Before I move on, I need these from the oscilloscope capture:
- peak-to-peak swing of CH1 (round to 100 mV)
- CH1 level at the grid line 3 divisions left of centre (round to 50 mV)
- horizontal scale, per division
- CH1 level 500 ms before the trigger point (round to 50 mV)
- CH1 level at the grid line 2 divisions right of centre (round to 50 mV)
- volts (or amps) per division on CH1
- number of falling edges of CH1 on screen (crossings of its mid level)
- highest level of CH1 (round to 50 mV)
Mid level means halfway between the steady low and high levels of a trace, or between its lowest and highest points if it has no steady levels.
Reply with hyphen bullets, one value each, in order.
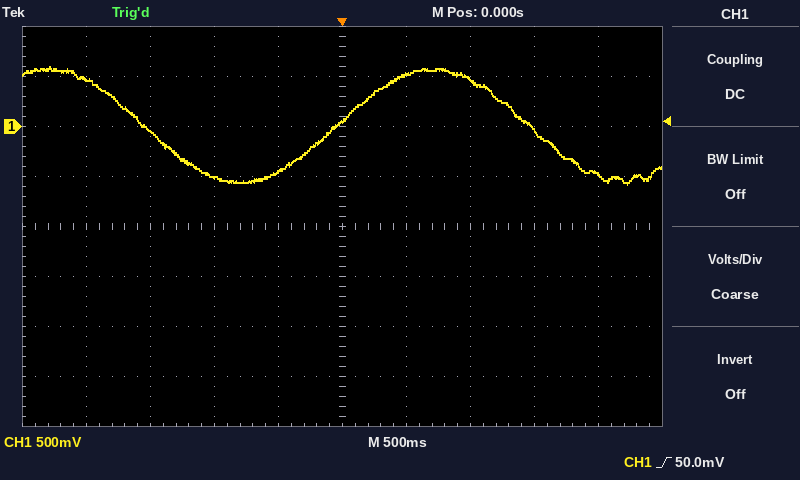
- 1.20 V
- -50 mV
- 500 ms
- -450 mV
- 450 mV
- 500 mV
- 2
- 600 mV
